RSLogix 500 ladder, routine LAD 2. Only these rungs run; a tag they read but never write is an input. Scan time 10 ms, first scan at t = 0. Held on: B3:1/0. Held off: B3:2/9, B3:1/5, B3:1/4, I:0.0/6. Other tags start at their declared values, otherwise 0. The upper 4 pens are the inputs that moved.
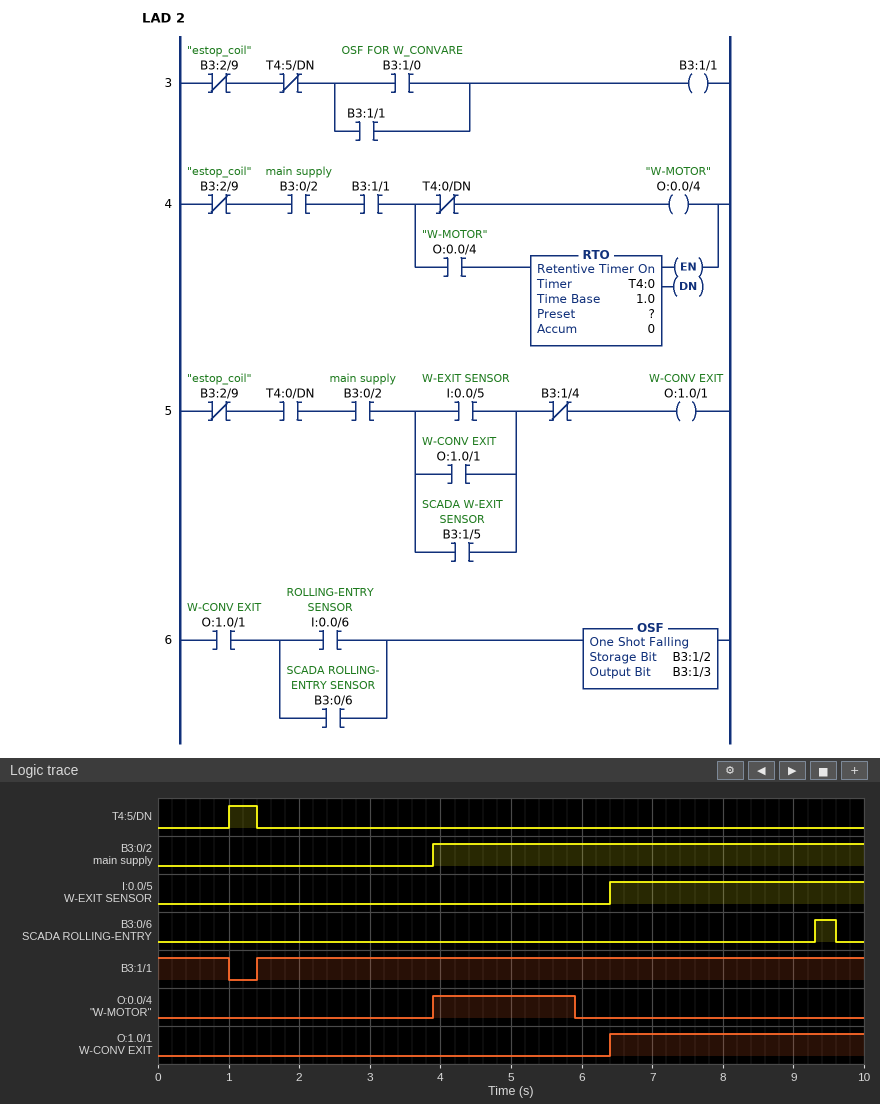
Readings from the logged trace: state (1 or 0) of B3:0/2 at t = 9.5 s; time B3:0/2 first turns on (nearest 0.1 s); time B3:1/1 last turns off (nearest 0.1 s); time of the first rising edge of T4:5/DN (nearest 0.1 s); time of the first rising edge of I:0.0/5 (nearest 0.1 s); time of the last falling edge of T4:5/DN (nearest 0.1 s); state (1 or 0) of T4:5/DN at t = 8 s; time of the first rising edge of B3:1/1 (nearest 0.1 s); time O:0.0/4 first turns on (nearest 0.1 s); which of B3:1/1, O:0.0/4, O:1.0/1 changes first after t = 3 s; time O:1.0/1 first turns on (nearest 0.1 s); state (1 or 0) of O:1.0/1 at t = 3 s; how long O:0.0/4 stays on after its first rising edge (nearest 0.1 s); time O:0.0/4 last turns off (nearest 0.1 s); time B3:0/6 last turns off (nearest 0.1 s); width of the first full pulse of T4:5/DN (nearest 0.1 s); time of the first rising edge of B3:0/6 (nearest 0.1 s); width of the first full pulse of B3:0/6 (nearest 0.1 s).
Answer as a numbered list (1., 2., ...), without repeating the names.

1. 1
2. 3.9 s
3. 1.0 s
4. 1.0 s
5. 6.4 s
6. 1.4 s
7. 0
8. 1.4 s
9. 3.9 s
10. O:0.0/4
11. 6.4 s
12. 0
13. 2.0 s
14. 5.9 s
15. 9.6 s
16. 0.4 s
17. 9.3 s
18. 0.3 s
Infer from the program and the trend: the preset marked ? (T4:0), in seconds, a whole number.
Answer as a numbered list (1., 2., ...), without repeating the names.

1. 2 s
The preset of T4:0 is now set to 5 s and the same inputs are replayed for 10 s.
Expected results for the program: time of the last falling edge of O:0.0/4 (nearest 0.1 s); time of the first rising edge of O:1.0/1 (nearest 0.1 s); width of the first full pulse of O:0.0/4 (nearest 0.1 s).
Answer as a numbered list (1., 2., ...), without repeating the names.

1. 8.9 s
2. 8.9 s
3. 5.0 s
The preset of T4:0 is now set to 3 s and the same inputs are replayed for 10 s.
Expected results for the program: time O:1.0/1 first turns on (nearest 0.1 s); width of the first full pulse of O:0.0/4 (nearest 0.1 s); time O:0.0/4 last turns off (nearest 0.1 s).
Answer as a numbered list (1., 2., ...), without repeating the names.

1. 6.9 s
2. 3.0 s
3. 6.9 s
